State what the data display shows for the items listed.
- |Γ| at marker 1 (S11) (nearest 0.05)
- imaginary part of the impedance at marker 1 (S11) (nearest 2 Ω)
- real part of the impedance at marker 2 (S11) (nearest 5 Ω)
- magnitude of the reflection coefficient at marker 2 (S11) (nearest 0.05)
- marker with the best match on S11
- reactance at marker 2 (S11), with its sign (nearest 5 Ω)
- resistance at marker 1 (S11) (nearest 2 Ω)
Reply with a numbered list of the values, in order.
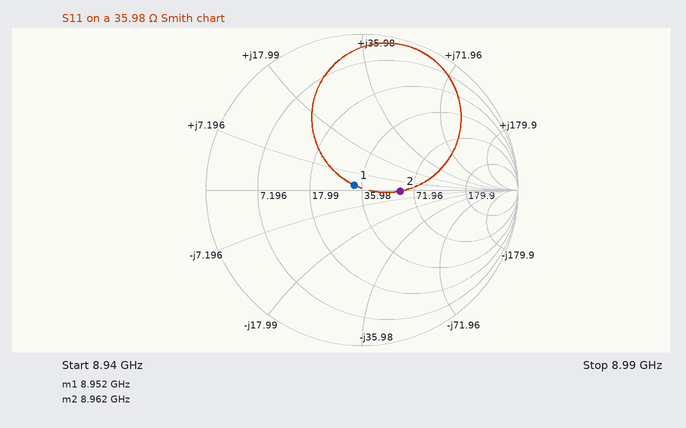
1. 0.05
2. +2 Ω
3. 60 Ω
4. 0.25
5. marker 1
6. 0 Ω
7. 32 Ω
